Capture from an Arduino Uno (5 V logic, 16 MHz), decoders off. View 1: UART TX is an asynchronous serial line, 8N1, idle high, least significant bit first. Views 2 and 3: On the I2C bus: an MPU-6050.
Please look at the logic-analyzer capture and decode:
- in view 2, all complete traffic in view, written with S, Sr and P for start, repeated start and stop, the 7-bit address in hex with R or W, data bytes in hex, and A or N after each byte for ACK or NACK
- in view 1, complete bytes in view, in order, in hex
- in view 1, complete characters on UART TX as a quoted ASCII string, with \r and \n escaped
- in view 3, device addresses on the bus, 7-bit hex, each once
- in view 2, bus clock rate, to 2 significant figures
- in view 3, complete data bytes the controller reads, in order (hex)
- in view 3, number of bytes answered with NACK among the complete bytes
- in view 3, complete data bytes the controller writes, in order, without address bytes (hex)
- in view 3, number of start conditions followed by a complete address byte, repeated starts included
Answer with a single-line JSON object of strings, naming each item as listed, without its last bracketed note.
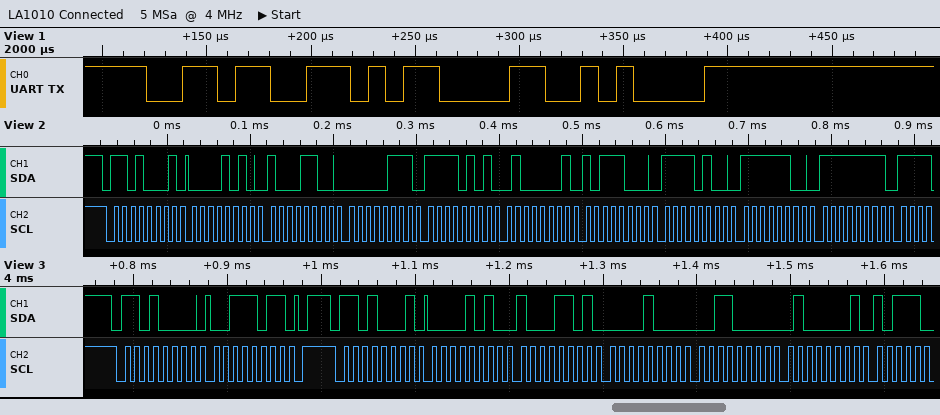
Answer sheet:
{"in view 2, all complete traffic in view, written with S, Sr and P for start, repeated start and stop, the 7-bit address in hex with R or W, data bytes in hex, and A or N after each byte for ACK or NACK": "S 68R A 0A A 8C A 07 A F5 A 41 A B8 A F4 A FC A FF A", "in view 1, complete bytes in view, in order, in hex": "36 0D 0A", "in view 1, complete characters on UART TX as a quoted ASCII string, with \\r and \\n escaped": "\"6\\r\\n\"", "in view 3, device addresses on the bus, 7-bit hex, each once": "0x68", "in view 2, bus clock rate, to 2 significant figures": "100 kHz", "in view 3, complete data bytes the controller reads, in order": "0A 8D 08 30 41", "in view 3, number of bytes answered with NACK among the complete bytes": "0", "in view 3, complete data bytes the controller writes, in order, without address bytes": "3B", "in view 3, number of start conditions followed by a complete address byte, repeated starts included": "2"}
